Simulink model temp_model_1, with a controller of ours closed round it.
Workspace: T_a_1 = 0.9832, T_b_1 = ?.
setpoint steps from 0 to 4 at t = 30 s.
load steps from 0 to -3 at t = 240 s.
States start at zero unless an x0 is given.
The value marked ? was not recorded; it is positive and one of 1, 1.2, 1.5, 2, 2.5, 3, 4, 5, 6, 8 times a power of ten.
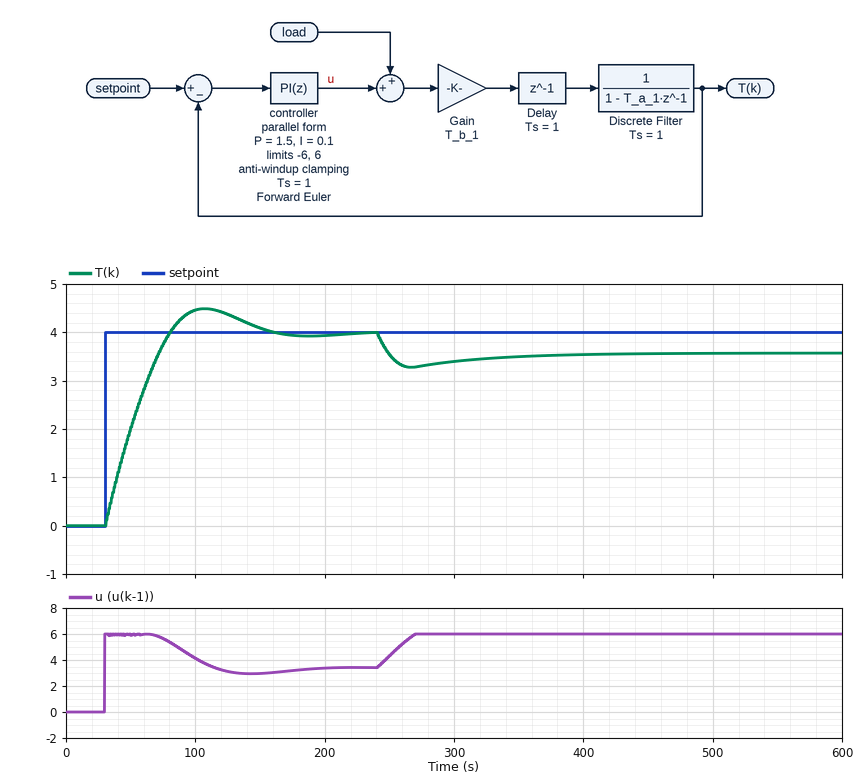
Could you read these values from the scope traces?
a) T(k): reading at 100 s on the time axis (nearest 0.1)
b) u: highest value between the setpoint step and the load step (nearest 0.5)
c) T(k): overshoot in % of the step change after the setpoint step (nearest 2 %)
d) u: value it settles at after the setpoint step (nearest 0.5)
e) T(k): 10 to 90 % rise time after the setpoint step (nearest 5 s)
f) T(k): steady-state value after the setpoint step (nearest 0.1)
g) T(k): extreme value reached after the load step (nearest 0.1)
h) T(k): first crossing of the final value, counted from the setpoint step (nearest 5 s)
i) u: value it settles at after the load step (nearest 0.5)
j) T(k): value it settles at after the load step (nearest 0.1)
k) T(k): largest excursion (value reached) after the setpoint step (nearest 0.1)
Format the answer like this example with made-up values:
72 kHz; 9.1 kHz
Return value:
4.5; 6.0; 12 %; 3.5; 40 s; 4.0; 3.3; 50 s; 6.0; 3.6; 4.5
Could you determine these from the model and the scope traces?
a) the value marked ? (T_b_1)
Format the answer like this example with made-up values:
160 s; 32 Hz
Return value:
0.02
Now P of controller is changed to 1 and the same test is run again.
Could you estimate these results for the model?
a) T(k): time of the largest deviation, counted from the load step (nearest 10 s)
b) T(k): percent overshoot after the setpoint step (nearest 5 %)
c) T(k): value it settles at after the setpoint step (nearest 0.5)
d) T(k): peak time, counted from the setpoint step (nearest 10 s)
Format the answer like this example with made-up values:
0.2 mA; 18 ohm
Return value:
30 s; 15 %; 4.0; 80 s
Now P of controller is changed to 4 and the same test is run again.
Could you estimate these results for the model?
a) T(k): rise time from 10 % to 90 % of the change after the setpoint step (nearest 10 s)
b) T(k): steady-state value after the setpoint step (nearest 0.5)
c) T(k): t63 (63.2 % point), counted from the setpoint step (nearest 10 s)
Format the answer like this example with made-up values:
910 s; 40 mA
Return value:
50 s; 4.0; 30 s
